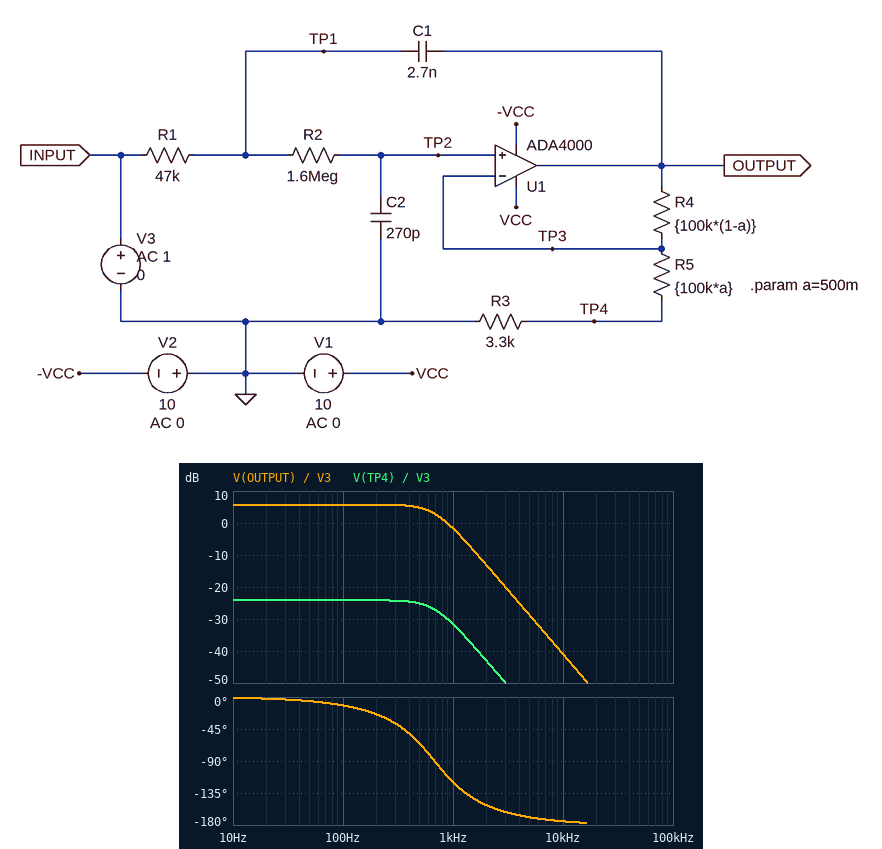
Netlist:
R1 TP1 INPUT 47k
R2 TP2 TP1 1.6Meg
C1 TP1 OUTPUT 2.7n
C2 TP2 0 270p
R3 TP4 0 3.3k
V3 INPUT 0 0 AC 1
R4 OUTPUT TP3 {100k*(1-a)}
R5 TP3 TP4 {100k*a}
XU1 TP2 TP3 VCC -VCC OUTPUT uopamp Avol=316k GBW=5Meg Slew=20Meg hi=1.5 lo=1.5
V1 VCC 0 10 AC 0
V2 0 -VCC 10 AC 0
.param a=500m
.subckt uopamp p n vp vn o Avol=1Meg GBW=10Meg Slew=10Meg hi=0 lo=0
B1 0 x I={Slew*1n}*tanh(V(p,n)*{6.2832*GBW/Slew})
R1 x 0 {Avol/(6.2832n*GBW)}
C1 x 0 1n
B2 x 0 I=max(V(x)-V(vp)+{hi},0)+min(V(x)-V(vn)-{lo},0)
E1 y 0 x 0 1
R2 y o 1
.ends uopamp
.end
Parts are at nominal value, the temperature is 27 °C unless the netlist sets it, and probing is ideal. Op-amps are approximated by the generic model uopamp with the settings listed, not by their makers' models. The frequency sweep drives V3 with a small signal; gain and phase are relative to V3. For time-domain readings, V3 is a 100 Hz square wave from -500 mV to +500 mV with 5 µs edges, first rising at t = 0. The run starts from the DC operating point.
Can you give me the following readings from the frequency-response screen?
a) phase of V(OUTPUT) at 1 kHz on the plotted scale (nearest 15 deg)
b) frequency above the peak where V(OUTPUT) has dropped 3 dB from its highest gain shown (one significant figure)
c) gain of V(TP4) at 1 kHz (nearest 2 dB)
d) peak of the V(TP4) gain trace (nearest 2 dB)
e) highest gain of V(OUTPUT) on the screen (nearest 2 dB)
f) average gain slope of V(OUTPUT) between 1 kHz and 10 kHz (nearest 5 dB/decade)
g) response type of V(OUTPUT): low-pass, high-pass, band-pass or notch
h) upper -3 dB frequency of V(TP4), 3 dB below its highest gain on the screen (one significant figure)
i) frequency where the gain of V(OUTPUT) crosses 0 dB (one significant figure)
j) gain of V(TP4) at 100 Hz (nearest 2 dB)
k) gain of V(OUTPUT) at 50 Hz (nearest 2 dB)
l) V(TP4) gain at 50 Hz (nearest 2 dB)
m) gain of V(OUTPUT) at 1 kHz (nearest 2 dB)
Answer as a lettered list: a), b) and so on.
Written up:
a) -120 deg
b) 700 Hz
c) -32 dB
d) -24 dB
e) 6 dB
f) -40 dB/decade
g) low-pass
h) 700 Hz
i) 900 Hz
j) -24 dB
k) 6 dB
l) -24 dB
m) -2 dB
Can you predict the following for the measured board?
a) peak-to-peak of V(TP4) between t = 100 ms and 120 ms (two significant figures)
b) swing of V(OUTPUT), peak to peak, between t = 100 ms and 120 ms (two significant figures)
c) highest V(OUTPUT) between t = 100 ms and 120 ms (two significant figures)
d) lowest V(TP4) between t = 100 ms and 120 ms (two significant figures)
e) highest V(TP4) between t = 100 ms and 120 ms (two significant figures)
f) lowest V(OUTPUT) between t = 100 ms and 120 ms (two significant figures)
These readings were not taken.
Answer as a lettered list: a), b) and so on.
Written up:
a) 68 mV
b) 2.1 V
c) 1.1 V
d) -34 mV
e) 34 mV
f) -1.1 V
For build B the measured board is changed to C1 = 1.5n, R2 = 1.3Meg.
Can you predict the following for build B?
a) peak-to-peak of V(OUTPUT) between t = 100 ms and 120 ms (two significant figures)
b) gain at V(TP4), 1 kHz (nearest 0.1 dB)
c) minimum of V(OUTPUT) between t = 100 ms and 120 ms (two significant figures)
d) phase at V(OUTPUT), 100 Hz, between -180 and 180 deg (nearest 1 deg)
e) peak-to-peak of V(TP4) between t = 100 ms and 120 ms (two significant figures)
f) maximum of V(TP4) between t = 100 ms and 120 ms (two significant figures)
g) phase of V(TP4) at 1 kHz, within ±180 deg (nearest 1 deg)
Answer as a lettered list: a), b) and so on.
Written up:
a) 1.9 V
b) -29.6 dB
c) -970 mV
d) -11 deg
e) 62 mV
f) 31 mV
g) -89 deg
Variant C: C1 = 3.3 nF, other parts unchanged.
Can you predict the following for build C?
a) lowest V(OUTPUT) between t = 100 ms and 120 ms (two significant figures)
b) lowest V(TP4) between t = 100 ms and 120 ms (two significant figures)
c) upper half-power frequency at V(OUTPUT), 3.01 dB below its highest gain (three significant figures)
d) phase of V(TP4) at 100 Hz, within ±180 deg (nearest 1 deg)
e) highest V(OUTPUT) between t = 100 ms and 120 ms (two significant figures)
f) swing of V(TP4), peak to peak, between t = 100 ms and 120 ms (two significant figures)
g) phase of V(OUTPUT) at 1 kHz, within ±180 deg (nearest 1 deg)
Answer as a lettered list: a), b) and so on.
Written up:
a) -1.2 V
b) -38 mV
c) 694 Hz
d) -11 deg
e) 1.2 V
f) 75 mV
g) -131 deg
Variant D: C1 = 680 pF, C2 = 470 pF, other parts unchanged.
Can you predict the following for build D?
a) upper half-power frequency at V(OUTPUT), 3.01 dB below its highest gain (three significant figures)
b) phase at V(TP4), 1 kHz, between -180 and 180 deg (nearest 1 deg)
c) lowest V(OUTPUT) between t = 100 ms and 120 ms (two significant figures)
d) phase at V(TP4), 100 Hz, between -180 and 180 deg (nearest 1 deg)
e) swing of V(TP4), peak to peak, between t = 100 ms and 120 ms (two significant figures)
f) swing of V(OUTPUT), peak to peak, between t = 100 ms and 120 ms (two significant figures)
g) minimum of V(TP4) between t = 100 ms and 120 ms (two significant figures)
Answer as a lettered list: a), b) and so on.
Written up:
a) 224 Hz
b) -89 deg
c) -970 mV
d) -25 deg
e) 62 mV
f) 1.9 V
g) -31 mV
